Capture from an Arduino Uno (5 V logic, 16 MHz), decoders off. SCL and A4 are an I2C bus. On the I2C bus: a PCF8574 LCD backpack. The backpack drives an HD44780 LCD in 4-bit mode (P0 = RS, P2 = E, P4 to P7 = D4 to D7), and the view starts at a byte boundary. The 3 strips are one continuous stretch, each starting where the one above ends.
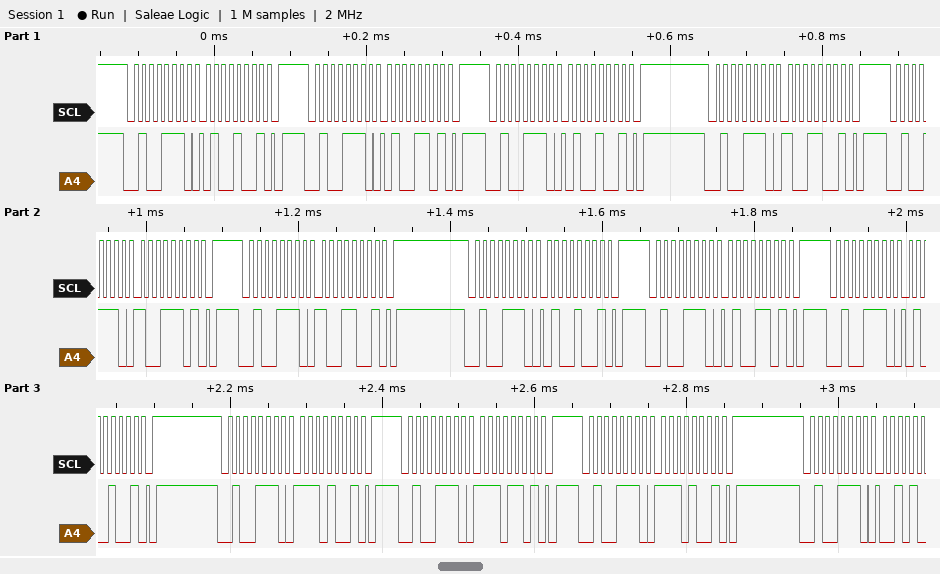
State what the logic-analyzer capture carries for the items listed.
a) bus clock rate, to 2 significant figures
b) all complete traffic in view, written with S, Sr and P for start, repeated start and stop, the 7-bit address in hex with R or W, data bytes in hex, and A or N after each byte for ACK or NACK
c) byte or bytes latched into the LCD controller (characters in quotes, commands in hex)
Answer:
100 kHz
S 27W A 49 A P S 27W A 4D A P S 27W A 49 A P S 27W A 99 A P S 27W A 9D A P S 27W A 99 A P S 27W A 49 A P S 27W A 4D A P S 27W A 49 A P S 27W A E9 A P S 27W A ED A P S 27W A E9 A P S 27W A
'I' 'N'
